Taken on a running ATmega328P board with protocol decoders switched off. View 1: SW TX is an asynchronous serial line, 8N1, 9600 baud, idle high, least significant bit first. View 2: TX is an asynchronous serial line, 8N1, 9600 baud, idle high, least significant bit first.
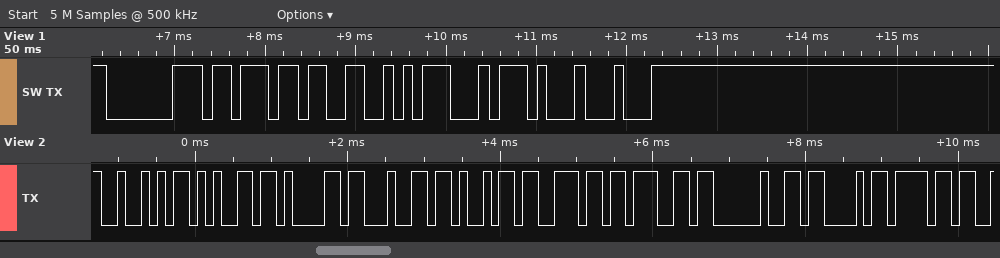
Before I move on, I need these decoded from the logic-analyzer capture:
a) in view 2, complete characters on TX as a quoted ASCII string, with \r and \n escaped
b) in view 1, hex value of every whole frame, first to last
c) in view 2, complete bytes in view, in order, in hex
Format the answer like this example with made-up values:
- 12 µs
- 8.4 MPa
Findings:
- "Reading Co"
- C0 BB 33 1D 17 C4
- 0x52 0x65 0x61 0x64 0x69 0x6E 0x67 0x20 0x43 0x6F
